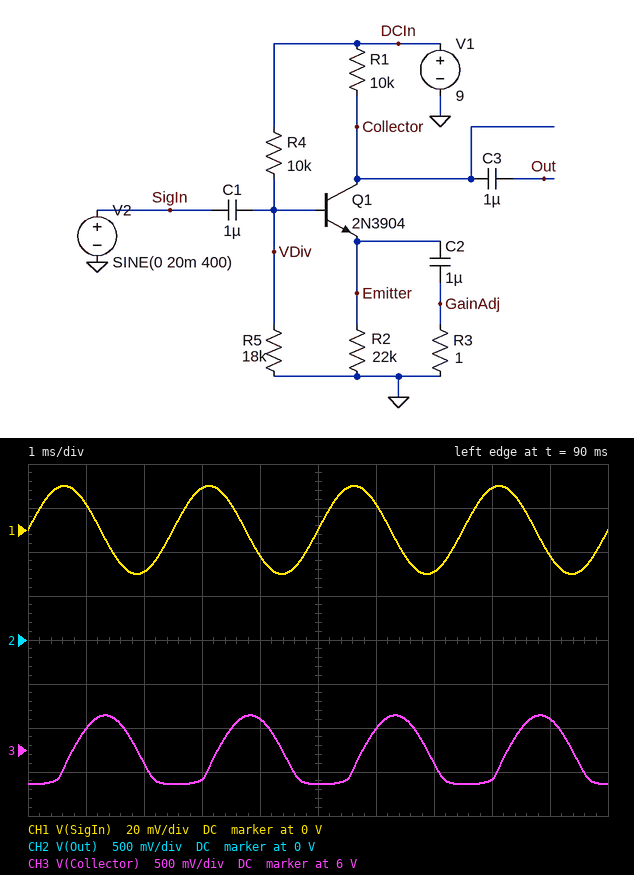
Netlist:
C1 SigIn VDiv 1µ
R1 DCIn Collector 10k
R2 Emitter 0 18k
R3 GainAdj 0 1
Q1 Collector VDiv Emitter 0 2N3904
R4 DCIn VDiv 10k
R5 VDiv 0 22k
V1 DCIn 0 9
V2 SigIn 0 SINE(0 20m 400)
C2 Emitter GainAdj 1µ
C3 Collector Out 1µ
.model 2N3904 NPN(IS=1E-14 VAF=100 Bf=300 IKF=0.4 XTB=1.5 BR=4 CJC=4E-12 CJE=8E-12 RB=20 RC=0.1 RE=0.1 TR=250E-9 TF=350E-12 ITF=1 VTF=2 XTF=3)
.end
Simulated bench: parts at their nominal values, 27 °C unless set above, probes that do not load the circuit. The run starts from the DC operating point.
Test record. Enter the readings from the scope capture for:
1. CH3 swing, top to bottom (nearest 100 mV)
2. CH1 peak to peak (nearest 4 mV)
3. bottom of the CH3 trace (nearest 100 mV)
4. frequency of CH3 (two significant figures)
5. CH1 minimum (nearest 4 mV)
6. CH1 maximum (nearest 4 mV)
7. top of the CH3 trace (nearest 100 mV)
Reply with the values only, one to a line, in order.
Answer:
800 mV
40 mV
5.6 V
400 Hz
-20 mV
20 mV
6.4 V
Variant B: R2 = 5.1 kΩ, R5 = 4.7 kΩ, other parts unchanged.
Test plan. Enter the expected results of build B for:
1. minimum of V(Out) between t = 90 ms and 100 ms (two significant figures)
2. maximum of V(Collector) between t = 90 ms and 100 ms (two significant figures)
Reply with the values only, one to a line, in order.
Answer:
4.1 V
5.1 V
